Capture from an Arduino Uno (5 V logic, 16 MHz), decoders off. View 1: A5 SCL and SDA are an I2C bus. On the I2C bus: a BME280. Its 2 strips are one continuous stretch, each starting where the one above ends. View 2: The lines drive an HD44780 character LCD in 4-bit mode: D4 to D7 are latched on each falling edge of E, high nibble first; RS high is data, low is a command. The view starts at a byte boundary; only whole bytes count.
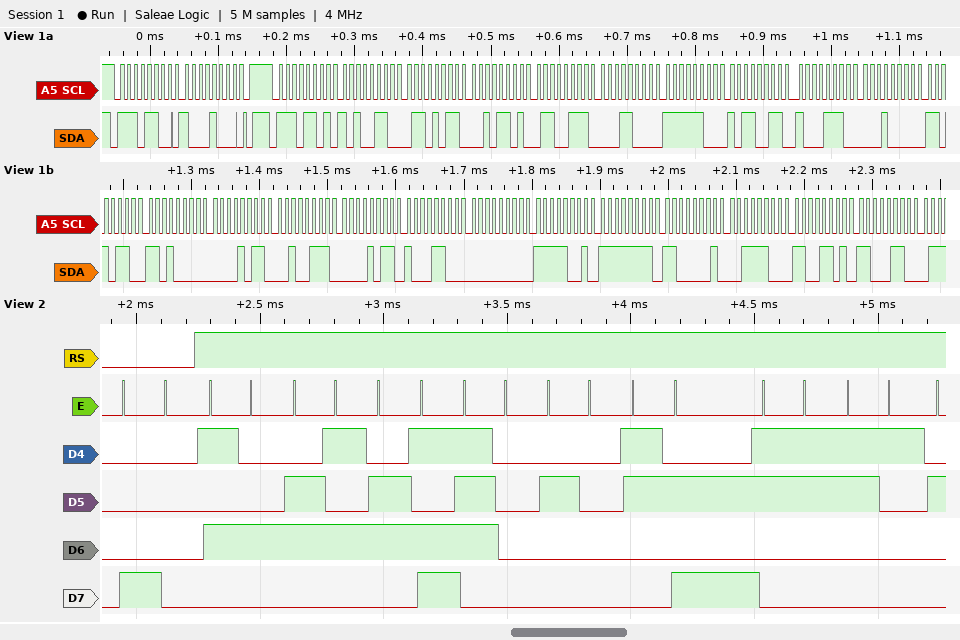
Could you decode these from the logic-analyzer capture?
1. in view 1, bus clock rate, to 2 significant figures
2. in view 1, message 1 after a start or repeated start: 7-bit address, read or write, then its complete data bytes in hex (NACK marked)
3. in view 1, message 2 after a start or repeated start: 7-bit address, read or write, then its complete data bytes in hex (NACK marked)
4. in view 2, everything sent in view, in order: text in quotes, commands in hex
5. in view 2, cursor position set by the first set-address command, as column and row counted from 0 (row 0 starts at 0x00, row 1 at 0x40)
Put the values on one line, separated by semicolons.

100 kHz; 0x76 write: 88; 0x76 read: A6 6B 2D 67 18 FC B3 8E 10 D6 D0 0B 27 0B 8C 00 F9 FF C1 3C CD C6; 0x80 "Temp :31"; column 0, row 0
